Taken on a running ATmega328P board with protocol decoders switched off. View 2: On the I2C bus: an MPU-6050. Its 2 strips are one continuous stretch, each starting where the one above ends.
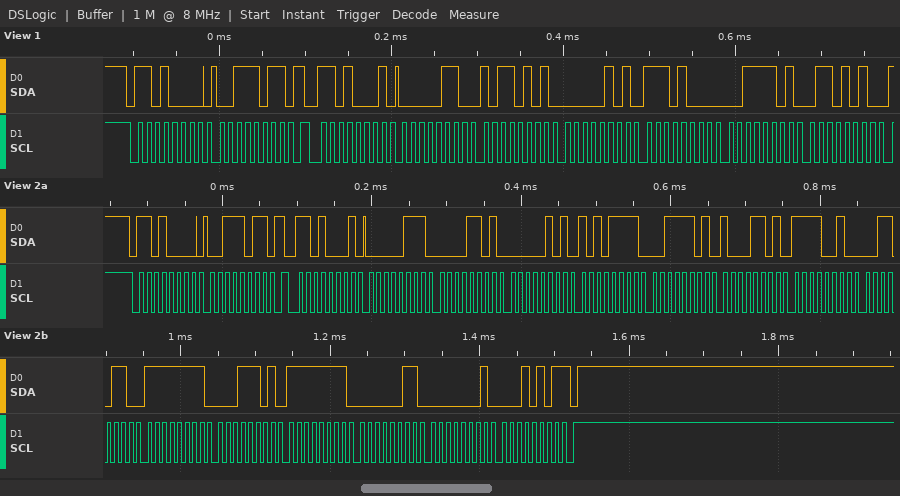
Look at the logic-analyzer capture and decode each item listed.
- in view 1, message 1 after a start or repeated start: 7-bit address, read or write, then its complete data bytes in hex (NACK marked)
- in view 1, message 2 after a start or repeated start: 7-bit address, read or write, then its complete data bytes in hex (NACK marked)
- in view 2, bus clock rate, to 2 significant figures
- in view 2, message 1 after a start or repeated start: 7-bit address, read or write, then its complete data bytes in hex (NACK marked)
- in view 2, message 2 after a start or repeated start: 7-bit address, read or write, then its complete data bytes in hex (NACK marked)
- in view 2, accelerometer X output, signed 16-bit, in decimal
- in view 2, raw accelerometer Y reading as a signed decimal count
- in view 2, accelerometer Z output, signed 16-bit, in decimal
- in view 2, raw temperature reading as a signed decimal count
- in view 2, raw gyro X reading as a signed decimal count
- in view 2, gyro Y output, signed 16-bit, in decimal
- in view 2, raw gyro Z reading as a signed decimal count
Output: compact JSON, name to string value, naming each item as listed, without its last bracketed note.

{"in view 1, message 1 after a start or repeated start: 7-bit address, read or write, then its complete data bytes in hex": "0x68 write: 3B", "in view 1, message 2 after a start or repeated start: 7-bit address, read or write, then its complete data bytes in hex": "0x68 read: 06 B5 05 E8 3D 6A", "in view 2, bus clock rate, to 2 significant figures": "100 kHz", "in view 2, message 1 after a start or repeated start: 7-bit address, read or write, then its complete data bytes in hex": "0x68 write: 3B", "in view 2, message 2 after a start or repeated start: 7-bit address, read or write, then its complete data bytes in hex": "0x68 read: 07 0D 05 AF 3D 8D F2 36 FF 1D FF 03 01 15 NACK", "in view 2, accelerometer X output, signed 16-bit, in decimal": "1805", "in view 2, raw accelerometer Y reading as a signed decimal count": "1455", "in view 2, accelerometer Z output, signed 16-bit, in decimal": "15757", "in view 2, raw temperature reading as a signed decimal count": "-3530", "in view 2, raw gyro X reading as a signed decimal count": "-227", "in view 2, gyro Y output, signed 16-bit, in decimal": "-253", "in view 2, raw gyro Z reading as a signed decimal count": "277"}
